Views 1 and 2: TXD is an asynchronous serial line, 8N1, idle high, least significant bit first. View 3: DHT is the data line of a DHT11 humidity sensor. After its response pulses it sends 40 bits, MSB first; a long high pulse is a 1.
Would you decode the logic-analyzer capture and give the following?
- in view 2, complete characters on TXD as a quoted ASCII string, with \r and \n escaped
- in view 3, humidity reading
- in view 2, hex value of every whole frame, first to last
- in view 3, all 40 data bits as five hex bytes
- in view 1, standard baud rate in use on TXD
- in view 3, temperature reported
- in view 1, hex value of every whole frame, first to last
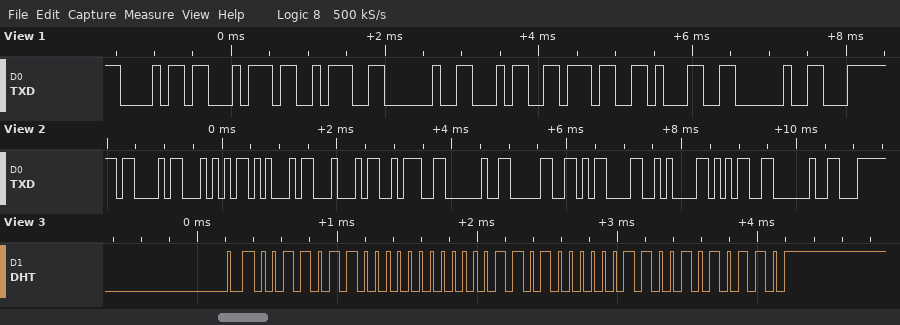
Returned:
"CTED: 0\r\n5 "
54 %
0x43 0x54 0x45 0x44 0x3A 0x20 0x30 0x0D 0x0A 0x35 0x20
36 00 1A 06 56
9600 baud
26.6 °C
68 74 3A 20 34 37 31 20
